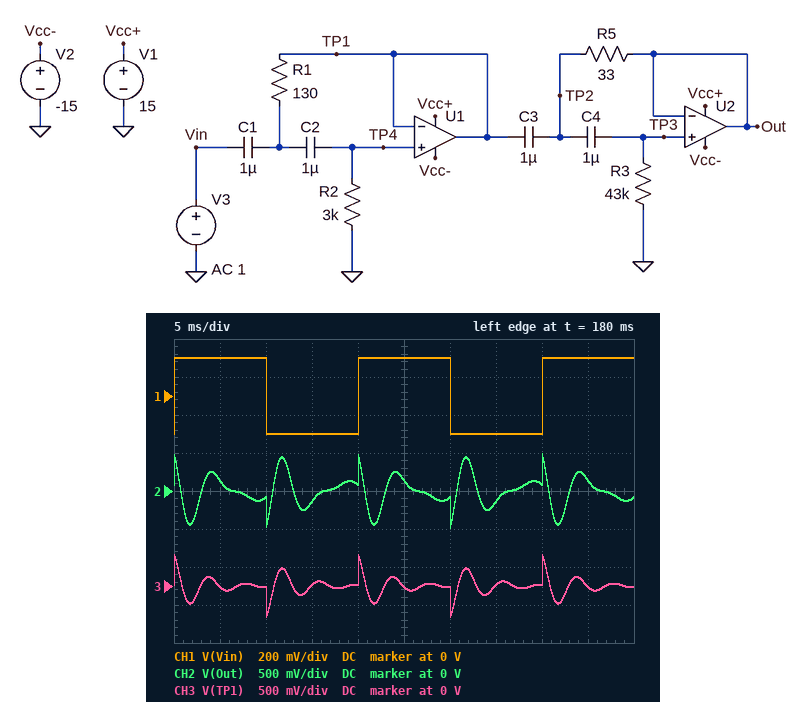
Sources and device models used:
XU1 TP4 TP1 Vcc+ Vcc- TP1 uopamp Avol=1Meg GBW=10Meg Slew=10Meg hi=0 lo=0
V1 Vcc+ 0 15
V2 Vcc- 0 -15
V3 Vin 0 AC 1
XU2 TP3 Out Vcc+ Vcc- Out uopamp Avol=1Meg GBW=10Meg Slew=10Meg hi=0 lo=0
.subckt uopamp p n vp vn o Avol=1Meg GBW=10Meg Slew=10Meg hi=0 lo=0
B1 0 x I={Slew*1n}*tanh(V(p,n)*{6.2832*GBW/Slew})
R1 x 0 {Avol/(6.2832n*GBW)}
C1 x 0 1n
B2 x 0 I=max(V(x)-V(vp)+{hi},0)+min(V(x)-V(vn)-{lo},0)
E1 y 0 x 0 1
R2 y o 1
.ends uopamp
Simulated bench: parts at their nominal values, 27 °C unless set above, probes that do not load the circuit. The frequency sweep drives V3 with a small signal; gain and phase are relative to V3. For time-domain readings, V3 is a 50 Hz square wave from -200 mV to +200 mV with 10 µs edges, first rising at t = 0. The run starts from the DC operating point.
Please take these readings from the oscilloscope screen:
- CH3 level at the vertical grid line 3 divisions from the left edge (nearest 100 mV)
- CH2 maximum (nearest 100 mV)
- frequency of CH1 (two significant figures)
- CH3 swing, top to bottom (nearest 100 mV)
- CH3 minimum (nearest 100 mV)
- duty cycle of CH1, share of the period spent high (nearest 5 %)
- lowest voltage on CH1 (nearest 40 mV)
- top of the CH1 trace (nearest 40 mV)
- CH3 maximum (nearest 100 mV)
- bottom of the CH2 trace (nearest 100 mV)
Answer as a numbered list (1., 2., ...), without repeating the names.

1. 0 V
2. 500 mV
3. 50 Hz
4. 800 mV
5. -400 mV
6. 50 %
7. -200 mV
8. 200 mV
9. 400 mV
10. -500 mV
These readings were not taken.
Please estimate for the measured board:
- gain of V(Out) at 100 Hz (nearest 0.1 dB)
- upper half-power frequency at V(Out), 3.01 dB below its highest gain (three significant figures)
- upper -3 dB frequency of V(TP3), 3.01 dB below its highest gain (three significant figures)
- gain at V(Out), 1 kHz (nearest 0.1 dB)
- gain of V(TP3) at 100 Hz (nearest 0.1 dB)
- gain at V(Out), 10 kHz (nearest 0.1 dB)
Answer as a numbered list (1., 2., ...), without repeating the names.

1. -12.9 dB
2. 138 Hz
3. 138 Hz
4. 0.7 dB
5. -12.9 dB
6. 0 dB
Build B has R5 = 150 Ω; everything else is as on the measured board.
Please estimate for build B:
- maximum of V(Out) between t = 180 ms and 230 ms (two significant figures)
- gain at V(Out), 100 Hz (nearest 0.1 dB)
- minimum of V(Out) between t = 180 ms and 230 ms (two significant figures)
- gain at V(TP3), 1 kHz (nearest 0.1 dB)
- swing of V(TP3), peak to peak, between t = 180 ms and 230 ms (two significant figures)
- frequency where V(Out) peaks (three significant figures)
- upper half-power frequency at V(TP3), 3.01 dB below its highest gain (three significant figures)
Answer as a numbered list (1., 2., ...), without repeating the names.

1. 420 mV
2. -10.7 dB
3. -420 mV
4. 0.6 dB
5. 840 mV
6. 265 Hz
7. 351 Hz
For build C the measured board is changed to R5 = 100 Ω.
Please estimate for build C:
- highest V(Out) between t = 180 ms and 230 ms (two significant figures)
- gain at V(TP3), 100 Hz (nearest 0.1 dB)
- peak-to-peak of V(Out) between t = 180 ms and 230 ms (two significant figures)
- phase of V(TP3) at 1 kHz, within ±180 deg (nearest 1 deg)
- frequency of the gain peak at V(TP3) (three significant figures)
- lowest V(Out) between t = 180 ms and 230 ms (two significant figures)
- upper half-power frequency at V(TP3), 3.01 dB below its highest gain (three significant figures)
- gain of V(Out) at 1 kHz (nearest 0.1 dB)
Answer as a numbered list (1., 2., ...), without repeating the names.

1. 430 mV
2. -7.4 dB
3. 860 mV
4. 7 deg
5. 264 Hz
6. -430 mV
7. 348 Hz
8. 0.6 dB
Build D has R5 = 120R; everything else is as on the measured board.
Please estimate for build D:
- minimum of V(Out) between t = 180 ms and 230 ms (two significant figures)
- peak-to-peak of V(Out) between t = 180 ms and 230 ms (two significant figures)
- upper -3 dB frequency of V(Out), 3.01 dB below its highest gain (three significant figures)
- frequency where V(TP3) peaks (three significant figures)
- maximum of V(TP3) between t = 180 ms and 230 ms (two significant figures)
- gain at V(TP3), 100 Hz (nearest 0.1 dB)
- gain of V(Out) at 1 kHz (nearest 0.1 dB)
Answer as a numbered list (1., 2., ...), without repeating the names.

1. -430 mV
2. 850 mV
3. 350 Hz
4. 265 Hz
5. 430 mV
6. -9.2 dB
7. 0.6 dB
